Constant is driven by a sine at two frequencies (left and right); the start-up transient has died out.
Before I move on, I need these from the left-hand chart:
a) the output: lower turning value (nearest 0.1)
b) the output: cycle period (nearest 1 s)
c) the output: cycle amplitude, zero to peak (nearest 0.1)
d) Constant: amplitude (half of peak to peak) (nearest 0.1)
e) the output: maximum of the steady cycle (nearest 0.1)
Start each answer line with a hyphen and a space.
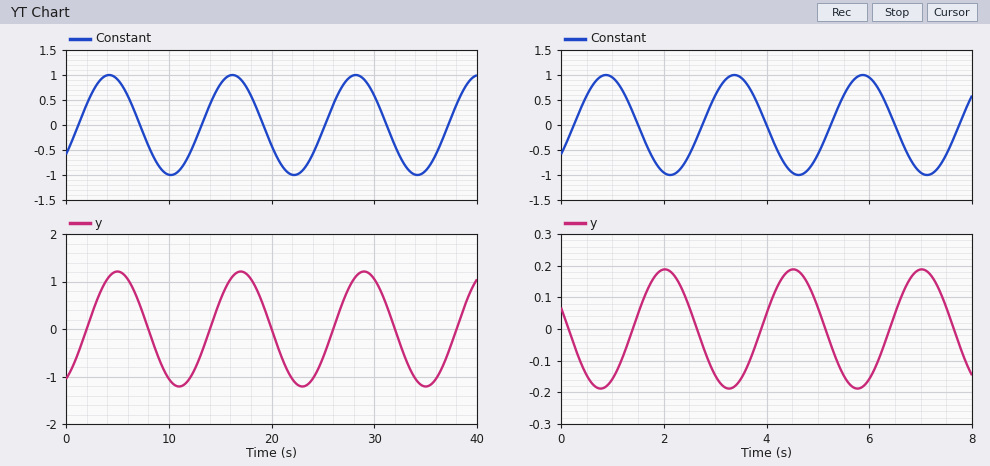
- -1.2
- 12 s
- 1.2
- 1.0
- 1.2
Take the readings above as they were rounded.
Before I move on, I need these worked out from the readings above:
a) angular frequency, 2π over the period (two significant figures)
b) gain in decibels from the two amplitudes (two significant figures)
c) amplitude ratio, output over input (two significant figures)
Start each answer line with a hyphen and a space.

- 0.52 rad/s
- 1.6 dB
- 1.2
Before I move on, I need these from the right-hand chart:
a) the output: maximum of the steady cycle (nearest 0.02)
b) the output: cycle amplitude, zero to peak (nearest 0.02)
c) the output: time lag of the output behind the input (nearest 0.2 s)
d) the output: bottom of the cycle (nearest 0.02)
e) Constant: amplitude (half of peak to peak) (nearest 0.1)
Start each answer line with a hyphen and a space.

- 0.18
- 0.18
- 1.2 s
- -0.18
- 1.0
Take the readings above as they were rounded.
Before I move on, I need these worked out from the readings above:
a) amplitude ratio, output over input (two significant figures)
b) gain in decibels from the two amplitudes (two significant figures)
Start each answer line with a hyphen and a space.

- 0.18
- -15 dB
